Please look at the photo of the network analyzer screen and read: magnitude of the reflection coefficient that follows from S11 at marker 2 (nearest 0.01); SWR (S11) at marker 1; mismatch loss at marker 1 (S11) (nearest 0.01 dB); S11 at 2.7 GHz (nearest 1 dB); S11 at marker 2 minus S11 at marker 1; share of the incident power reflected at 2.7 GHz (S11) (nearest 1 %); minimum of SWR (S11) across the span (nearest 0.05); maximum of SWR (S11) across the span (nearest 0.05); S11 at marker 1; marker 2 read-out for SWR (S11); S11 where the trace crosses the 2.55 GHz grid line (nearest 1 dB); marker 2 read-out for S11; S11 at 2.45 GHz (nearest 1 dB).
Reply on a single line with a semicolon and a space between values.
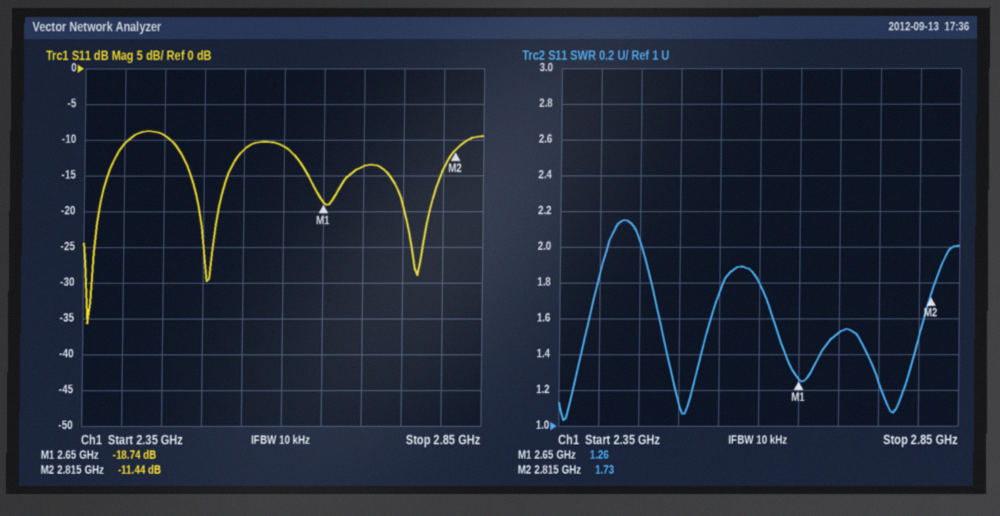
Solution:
0.27; 1.26; 0.06 dB; -14 dB; 7.30 dB; 4 %; 1.05; 2.15; -18.74 dB; 1.73; -11 dB; -11.44 dB; -9 dB
